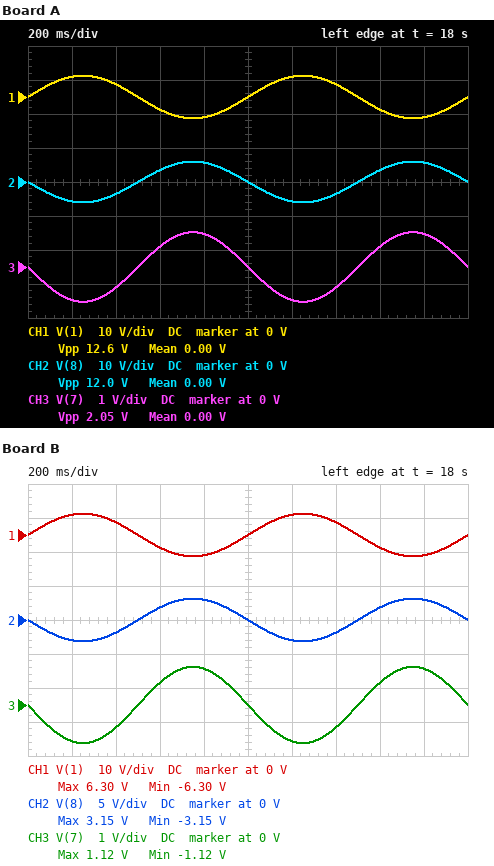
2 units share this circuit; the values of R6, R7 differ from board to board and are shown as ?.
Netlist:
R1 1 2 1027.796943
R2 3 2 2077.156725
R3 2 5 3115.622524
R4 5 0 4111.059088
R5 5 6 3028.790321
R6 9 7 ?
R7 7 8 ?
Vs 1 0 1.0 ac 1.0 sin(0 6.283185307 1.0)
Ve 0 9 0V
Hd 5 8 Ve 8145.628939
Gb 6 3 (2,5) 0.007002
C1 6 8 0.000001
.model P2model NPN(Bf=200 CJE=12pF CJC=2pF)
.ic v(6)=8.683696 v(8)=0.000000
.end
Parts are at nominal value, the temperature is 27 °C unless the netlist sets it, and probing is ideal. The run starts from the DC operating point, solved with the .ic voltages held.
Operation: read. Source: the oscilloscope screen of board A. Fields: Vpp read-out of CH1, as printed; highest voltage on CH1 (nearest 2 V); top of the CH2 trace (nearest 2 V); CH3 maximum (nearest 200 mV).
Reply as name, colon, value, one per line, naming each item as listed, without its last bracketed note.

Vpp read-out of CH1, as printed: 12.6 V
highest voltage on CH1: 6 V
top of the CH2 trace: 6 V
CH3 maximum: 1.0 V
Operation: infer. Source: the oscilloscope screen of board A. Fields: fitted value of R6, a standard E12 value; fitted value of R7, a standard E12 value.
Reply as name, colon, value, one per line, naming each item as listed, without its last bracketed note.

fitted value of R6, a standard E12 value: 680 Ω
fitted value of R7, a standard E12 value: 3.3 kΩ
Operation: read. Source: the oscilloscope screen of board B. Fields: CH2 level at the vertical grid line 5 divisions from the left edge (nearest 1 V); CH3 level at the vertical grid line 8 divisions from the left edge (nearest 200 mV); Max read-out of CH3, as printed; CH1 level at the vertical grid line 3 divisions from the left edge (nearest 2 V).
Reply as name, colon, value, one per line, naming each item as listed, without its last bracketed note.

CH2 level at the vertical grid line 5 divisions from the left edge: 0 V
CH3 level at the vertical grid line 8 divisions from the left edge: 600 mV
Max read-out of CH3, as printed: 1.12 V
CH1 level at the vertical grid line 3 divisions from the left edge: -4 V
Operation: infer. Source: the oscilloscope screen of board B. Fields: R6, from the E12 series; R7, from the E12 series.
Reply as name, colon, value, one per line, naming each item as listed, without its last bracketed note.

R6, from the E12 series: 1 kΩ
R7, from the E12 series: 1.8 kΩ
